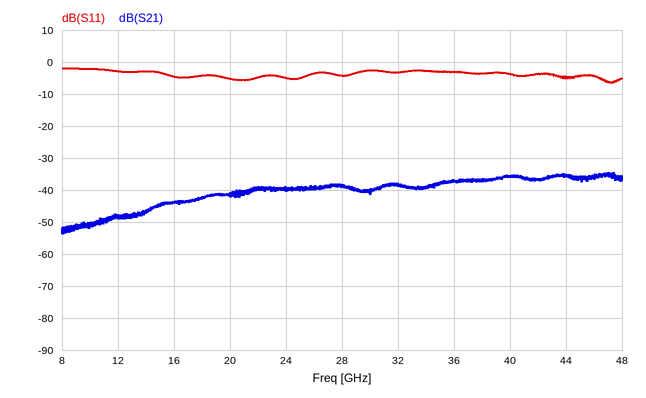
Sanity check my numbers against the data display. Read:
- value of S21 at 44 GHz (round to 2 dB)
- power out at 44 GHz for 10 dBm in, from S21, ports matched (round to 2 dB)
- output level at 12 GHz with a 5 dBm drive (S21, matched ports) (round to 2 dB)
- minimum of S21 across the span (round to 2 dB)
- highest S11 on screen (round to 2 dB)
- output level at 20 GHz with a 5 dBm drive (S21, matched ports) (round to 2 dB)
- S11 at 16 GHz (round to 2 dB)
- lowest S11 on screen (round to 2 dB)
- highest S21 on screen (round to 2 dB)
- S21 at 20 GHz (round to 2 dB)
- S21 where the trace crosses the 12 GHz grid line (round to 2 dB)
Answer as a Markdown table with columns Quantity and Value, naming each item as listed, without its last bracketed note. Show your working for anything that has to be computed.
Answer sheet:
| Quantity | Value |
|---|---|
| value of S21 at 44 GHz | -36 dB |
| power out at 44 GHz for 10 dBm in, from S21, ports matched | 10 dBm + (-36 dB) = -26 dBm |
| output level at 12 GHz with a 5 dBm drive (S21, matched ports) | 5 dBm + (-48 dB) = -44 dBm |
| minimum of S21 across the span | -54 dB |
| highest S11 on screen | -2 dB |
| output level at 20 GHz with a 5 dBm drive (S21, matched ports) | 5 dBm + (-42 dB) = -36 dBm |
| S11 at 16 GHz | -4 dB |
| lowest S11 on screen | -6 dB |
| highest S21 on screen | -34 dB |
| S21 at 20 GHz | -42 dB |
| S21 where the trace crosses the 12 GHz grid line | -48 dB |
